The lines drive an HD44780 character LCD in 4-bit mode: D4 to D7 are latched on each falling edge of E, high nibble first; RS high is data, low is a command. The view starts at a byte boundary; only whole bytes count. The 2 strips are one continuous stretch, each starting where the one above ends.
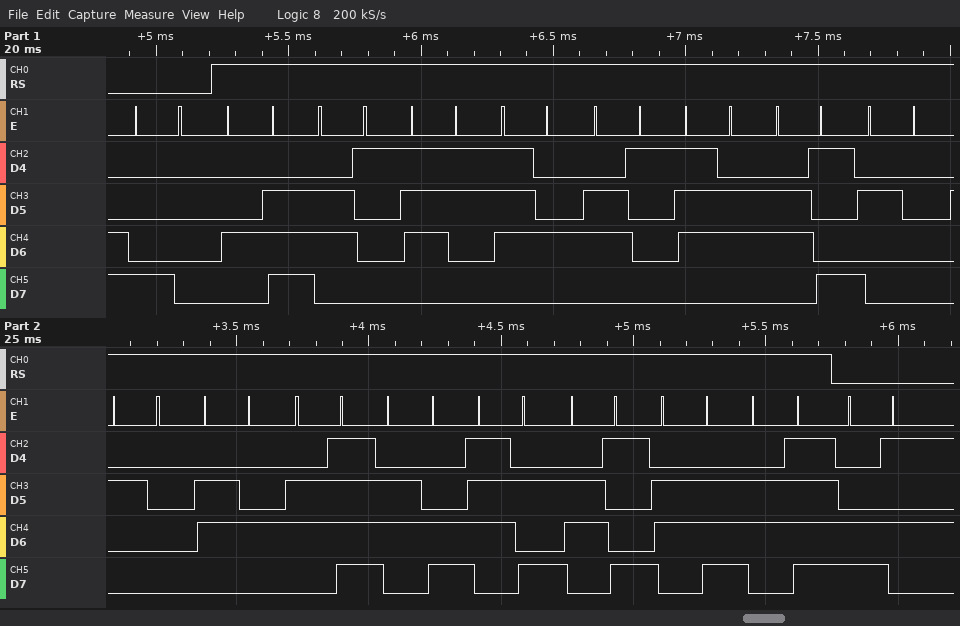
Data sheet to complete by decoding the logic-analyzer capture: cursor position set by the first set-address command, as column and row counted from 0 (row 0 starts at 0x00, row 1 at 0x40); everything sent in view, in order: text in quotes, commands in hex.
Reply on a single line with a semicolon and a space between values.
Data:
column 0, row 0; 0x80 "Nastavi  dolzino" 0xC5
